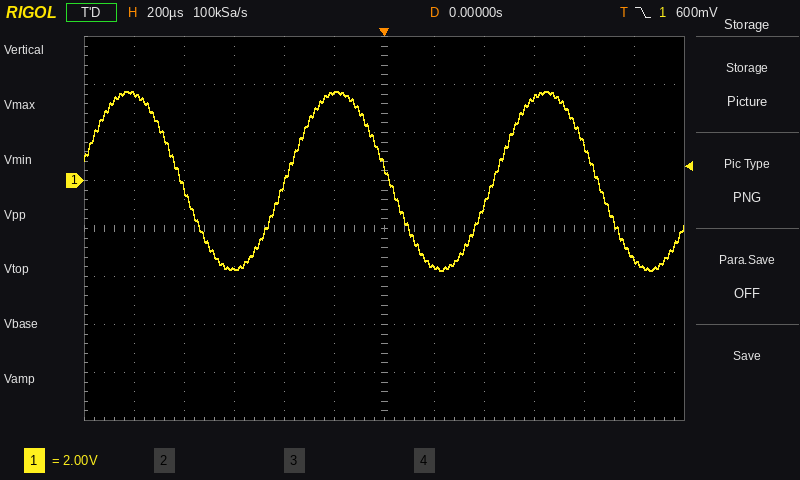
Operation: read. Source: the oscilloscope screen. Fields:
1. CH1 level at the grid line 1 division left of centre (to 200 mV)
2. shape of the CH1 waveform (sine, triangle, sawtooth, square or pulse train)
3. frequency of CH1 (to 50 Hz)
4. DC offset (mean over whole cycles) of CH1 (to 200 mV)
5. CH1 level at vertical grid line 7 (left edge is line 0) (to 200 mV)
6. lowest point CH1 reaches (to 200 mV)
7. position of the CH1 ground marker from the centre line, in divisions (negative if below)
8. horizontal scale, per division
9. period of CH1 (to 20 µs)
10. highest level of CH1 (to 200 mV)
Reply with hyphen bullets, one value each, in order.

- 3.6 V
- sine
- 1.20 kHz
- 0.0 V
- -3.6 V
- -3.8 V
- +1.0 div
- 200 µs
- 840 µs
- 3.8 V
